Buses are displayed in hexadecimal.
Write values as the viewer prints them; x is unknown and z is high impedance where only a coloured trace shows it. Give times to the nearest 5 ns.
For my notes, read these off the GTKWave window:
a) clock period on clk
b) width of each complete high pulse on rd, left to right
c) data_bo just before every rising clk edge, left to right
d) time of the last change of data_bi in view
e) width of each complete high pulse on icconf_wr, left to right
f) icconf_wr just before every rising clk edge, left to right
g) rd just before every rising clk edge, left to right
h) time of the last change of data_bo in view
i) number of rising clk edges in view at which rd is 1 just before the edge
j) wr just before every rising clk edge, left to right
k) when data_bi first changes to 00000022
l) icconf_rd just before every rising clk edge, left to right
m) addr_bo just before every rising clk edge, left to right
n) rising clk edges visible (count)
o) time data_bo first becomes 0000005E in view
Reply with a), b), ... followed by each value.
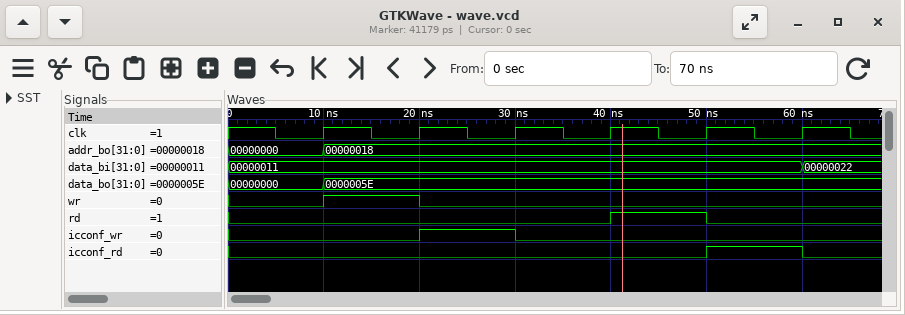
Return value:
a) 10 ns
b) 10 ns
c) 00000000, 0000005E, 0000005E, 0000005E, 0000005E, 0000005E
d) 60 ns
e) 10 ns
f) 0 0 1 0 0 0
g) 0 0 0 0 1 0
h) 10 ns
i) 1
j) 0 1 0 0 0 0
k) 60 ns
l) 0 0 0 0 0 1
m) 00000000, 00000018, 00000018, 00000018, 00000018, 00000018
n) 6
o) 10 ns
